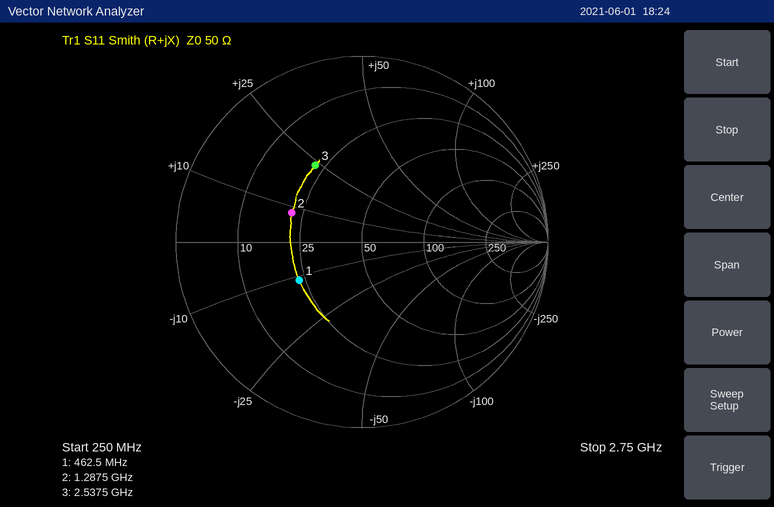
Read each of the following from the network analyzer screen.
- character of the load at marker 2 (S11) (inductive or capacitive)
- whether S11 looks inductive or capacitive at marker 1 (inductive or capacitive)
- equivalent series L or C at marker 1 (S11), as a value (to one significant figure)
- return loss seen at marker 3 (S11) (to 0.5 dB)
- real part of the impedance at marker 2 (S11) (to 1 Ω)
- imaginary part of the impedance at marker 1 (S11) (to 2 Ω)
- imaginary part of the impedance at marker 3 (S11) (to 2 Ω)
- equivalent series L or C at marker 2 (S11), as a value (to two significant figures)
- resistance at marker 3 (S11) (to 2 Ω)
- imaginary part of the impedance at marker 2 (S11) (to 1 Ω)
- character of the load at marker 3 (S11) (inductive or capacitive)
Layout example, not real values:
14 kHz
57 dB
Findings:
inductive
capacitive
30 pF
6.5 dB
22 Ω
-12 Ω
+24 Ω
1.0 nH
22 Ω
+8 Ω
inductive
